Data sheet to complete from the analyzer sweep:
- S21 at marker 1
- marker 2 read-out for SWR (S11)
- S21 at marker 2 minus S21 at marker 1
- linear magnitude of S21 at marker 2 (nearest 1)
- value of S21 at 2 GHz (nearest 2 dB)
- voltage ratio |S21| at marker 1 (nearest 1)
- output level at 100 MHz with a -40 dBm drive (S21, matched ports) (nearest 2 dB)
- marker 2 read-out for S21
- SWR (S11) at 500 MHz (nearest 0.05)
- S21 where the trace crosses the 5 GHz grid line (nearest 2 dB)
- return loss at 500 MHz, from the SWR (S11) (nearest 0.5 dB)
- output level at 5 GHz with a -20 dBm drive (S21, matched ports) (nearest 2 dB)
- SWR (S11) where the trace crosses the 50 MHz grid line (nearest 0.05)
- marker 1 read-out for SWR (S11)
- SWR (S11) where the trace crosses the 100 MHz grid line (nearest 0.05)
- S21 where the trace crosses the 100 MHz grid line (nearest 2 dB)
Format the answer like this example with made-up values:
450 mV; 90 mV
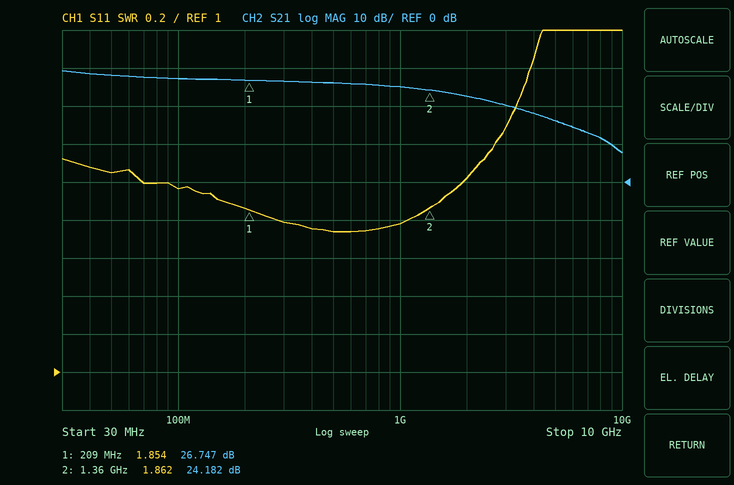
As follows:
26.747 dB; 1.862; -2.565 dB; 16; 22 dB; 22; -12 dBm; 24.182 dB; 1.75; 16 dB; 11.5 dB; -4 dBm; 2.05; 1.854; 1.95; 28 dB
